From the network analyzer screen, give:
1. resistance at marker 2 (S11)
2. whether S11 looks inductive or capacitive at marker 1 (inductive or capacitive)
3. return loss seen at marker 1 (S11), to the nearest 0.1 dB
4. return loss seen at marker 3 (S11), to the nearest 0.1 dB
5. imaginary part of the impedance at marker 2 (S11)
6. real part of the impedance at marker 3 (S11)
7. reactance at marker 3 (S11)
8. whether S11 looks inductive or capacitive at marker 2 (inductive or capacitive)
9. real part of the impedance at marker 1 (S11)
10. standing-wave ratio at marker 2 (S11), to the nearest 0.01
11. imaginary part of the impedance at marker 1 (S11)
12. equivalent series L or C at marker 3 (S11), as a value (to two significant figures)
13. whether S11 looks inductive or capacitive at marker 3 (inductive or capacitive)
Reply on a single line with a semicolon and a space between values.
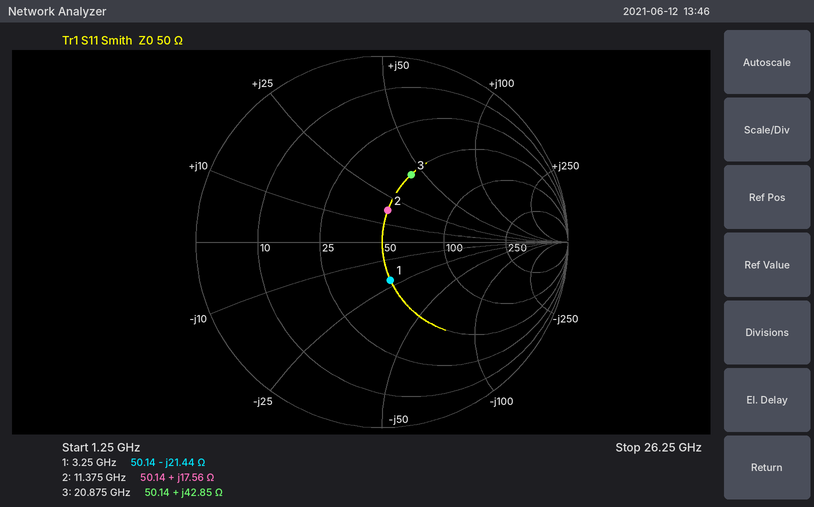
50.14 Ω; capacitive; 13.6 dB; 8.1 dB; +17.56 Ω; 50.14 Ω; +42.85 Ω; inductive; 50.14 Ω; 1.42; -21.44 Ω; 330 pH; inductive
